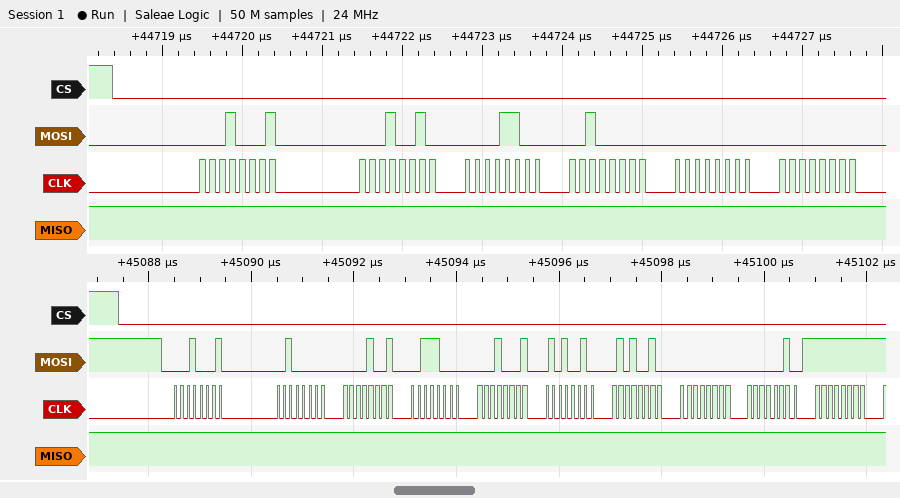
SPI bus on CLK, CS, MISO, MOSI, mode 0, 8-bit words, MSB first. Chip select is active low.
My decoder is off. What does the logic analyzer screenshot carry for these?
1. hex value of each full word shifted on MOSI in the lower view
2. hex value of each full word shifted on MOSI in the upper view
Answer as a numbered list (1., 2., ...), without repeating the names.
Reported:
1. 11, 20, 09, 38, 11, 52, 52, 00, 02, FF
2. 11, 12, 0C, 20, 00, 00
